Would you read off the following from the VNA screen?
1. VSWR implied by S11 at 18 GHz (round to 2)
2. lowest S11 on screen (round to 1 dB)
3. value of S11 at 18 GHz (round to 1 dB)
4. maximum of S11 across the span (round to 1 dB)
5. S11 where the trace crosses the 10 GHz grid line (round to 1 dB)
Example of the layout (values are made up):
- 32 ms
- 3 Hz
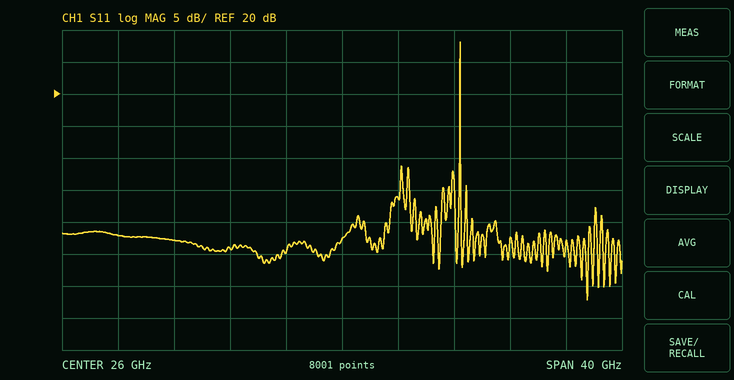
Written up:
- 4
- -12 dB
- -4 dB
- 28 dB
- -2 dB
